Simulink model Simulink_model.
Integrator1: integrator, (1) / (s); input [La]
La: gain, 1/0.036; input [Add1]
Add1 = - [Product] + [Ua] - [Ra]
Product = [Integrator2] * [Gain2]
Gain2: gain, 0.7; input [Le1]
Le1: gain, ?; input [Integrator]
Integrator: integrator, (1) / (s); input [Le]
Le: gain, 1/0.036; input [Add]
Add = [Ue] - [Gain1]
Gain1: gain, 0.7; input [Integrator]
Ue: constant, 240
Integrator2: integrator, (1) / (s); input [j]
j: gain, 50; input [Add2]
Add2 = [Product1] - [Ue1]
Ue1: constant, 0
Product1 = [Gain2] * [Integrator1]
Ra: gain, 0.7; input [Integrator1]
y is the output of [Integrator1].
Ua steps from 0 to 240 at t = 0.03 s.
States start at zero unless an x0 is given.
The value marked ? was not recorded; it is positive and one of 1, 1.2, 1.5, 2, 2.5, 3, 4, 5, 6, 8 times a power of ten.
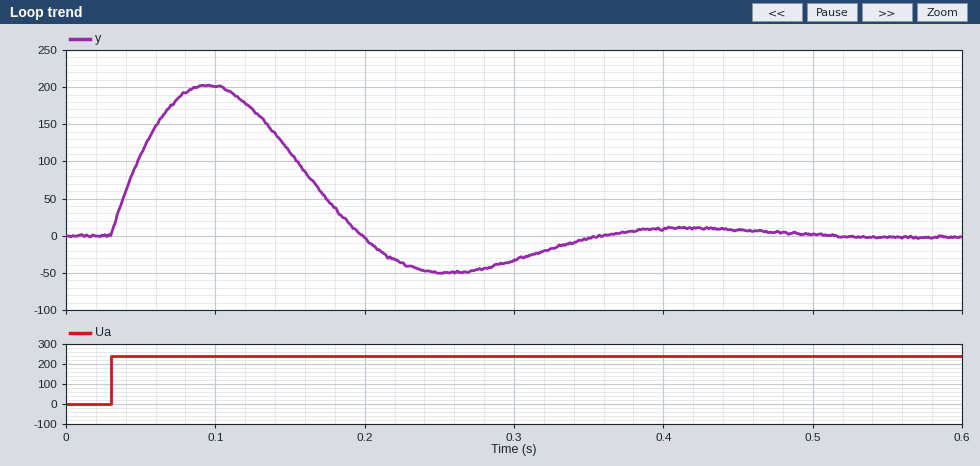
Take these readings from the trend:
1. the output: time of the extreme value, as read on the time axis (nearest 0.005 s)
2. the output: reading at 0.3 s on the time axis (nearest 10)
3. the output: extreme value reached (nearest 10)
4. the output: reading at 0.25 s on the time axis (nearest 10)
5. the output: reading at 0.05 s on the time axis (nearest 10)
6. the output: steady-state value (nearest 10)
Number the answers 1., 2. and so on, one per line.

1. 0.095 s
2. -30
3. 200
4. -50
5. 110
6. 0
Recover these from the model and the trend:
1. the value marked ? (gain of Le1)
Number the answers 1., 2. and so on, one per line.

1. 0.0025
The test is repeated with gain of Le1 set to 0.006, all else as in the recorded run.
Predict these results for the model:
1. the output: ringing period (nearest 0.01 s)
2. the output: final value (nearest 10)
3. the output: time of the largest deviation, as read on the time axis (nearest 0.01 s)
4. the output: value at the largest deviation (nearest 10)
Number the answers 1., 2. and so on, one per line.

1. 0.13 s
2. 0
3. 0.07 s
4. 130
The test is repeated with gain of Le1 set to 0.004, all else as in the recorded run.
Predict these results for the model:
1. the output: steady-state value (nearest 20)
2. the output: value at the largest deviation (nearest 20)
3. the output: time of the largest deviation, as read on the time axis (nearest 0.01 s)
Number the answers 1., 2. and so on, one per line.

1. 0
2. 160
3. 0.08 s
